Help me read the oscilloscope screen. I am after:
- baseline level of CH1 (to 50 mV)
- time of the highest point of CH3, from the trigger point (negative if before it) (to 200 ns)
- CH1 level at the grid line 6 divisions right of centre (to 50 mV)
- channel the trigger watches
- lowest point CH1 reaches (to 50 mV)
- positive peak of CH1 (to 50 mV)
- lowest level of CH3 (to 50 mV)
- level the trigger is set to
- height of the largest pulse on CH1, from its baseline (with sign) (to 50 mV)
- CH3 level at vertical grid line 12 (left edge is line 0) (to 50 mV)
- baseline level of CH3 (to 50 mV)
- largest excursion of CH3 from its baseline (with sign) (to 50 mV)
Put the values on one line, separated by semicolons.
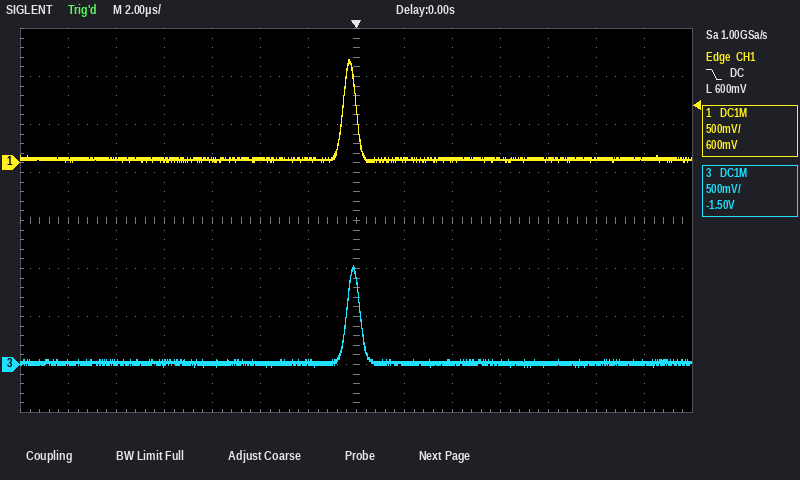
50 mV; -200 ns; 50 mV; CH1; 0 mV; 1.10 V; -50 mV; 600 mV; +1.05 V; 0 mV; 0 mV; +1.00 V
